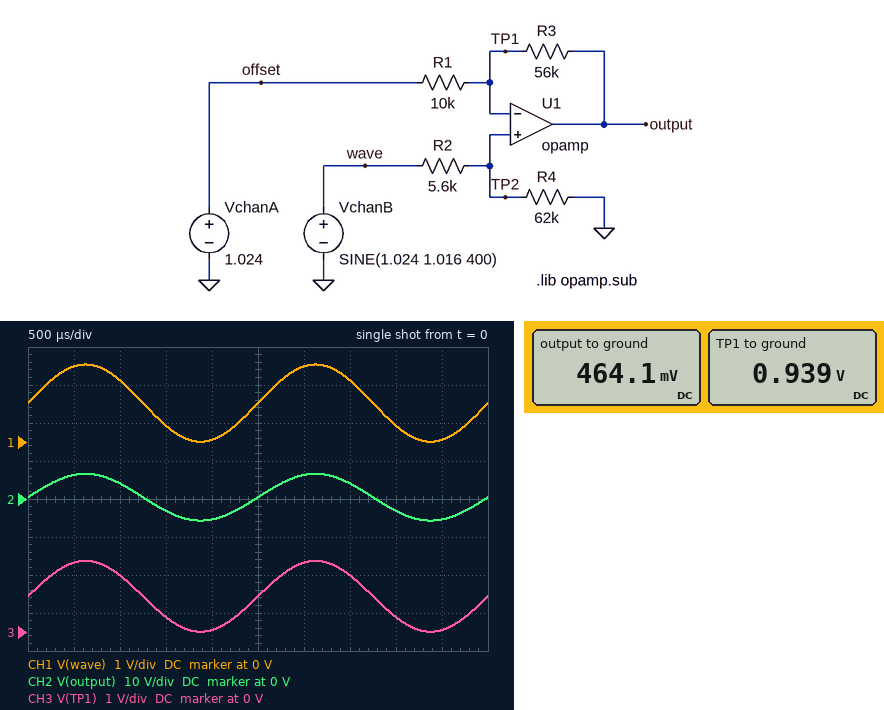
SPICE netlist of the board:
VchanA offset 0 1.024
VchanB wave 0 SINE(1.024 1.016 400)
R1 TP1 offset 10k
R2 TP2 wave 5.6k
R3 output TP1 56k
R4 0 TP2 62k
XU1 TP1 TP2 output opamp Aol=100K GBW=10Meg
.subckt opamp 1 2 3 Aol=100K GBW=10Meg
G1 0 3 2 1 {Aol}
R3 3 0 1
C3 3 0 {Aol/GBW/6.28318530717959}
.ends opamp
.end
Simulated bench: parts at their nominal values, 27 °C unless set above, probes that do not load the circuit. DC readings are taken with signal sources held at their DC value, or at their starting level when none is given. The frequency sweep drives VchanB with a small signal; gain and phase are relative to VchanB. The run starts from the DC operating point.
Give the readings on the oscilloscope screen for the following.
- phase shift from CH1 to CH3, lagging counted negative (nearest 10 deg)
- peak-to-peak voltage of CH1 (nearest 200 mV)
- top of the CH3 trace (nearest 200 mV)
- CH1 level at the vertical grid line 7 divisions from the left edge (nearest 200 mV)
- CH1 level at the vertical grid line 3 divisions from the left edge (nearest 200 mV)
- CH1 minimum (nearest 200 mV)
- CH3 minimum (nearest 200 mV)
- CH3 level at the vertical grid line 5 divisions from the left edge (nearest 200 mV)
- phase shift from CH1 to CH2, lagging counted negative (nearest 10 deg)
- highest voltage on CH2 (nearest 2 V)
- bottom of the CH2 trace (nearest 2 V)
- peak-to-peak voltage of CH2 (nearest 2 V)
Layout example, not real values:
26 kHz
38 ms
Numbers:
0 deg
2.0 V
1.8 V
1.6 V
400 mV
0 V
0 V
1.0 V
0 deg
6 V
-6 V
12 V
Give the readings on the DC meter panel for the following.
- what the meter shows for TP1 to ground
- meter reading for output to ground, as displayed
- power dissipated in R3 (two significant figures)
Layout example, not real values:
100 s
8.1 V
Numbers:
0.939 V
464.1 mV
4.0 µW
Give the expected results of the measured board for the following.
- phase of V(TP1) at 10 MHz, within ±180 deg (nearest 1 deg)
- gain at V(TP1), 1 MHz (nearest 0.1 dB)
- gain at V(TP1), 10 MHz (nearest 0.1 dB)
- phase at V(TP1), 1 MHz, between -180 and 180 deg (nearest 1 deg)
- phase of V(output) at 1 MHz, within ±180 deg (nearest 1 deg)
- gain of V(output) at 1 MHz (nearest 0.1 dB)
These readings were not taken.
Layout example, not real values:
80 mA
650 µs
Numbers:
-81 deg
-2.3 dB
-17.2 dB
-33 deg
-33 deg
14.1 dB
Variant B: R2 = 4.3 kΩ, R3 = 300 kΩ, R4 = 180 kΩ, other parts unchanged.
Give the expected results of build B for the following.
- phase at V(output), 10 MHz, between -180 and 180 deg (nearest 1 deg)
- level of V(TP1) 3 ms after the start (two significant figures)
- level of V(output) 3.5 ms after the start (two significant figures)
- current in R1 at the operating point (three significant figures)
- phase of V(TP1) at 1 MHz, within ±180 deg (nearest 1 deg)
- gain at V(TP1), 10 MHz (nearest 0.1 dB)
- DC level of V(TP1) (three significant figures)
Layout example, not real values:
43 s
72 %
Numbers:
-88 deg
1.9 V
18 V
2.39 µA
-72 deg
-30.0 dB
1.00 V
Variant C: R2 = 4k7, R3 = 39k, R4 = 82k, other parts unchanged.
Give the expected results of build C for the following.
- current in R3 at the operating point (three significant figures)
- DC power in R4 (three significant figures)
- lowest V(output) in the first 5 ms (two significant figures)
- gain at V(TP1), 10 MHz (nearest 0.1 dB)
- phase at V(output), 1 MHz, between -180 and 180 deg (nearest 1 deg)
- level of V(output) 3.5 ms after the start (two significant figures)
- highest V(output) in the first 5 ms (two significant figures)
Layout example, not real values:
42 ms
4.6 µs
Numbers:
5.55 µA
11.4 µW
-4.0 V
-14.5 dB
-26 deg
3.5 V
5.5 V
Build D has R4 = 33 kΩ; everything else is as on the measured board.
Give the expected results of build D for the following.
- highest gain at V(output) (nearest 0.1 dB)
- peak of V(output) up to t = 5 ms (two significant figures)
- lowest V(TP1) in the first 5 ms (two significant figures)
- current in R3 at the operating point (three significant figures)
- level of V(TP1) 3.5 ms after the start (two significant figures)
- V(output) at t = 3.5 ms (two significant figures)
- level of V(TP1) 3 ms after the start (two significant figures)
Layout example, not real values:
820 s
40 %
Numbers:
15.0 dB
5.8 V
6.9 mV
14.9 µA
1.4 V
3.4 V
1.7 V
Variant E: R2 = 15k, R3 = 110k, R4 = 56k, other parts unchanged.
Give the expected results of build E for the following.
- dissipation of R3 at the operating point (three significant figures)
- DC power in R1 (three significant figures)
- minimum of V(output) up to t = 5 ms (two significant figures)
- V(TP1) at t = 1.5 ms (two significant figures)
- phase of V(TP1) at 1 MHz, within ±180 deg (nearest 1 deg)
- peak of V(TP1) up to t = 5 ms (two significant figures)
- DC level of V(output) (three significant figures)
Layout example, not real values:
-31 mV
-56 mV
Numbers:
51.5 µW
4.68 µW
-11 V
340 mV
-50 deg
1.6 V
-1.57 V
